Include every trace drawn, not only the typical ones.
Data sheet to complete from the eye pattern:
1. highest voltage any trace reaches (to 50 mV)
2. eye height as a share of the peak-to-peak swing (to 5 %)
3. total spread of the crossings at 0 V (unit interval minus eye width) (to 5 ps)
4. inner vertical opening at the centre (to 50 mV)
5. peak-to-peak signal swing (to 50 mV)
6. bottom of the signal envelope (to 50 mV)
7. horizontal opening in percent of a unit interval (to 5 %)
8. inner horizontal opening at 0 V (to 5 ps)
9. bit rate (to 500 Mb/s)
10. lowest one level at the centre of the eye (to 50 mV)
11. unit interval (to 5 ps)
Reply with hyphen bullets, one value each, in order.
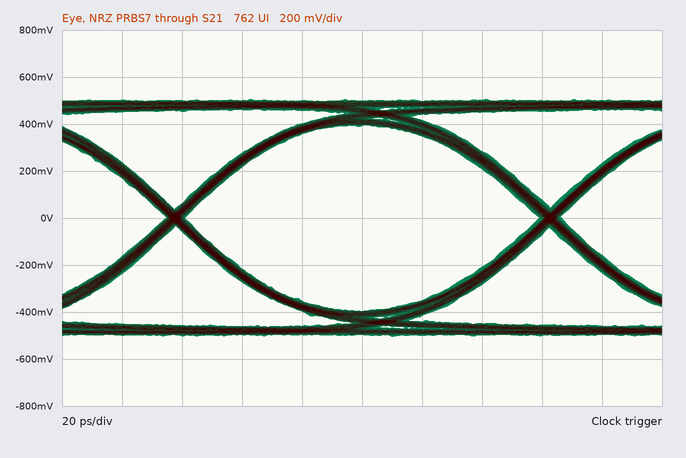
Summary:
- 500 mV
- 80 %
- 5 ps
- 800 mV
- 1.00 V
- -500 mV
- 95 %
- 120 ps
- 8.0 Gb/s
- 400 mV
- 125 ps
